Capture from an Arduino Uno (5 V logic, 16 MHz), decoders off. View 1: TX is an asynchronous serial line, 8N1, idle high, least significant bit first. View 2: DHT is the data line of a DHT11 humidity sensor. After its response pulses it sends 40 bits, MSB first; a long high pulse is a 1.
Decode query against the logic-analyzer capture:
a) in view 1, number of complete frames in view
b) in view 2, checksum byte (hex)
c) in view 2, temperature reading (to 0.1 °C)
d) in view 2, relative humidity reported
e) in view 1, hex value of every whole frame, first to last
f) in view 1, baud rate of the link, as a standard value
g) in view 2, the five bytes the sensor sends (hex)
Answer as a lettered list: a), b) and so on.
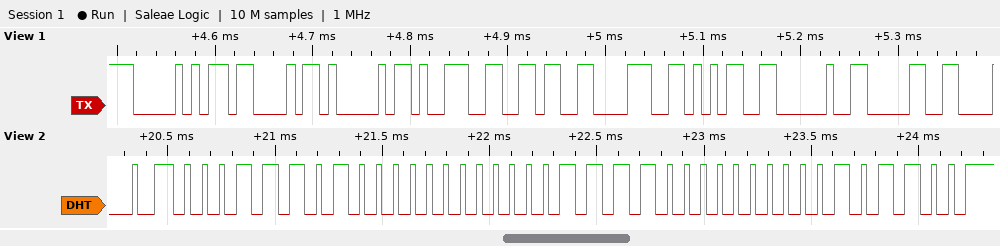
a) 9
b) 0x2C
c) 15.0 °C
d) 29 %
e) 50 43 41 39 36 38 35 20 30
f) 115200 baud
g) 1D 00 0F 00 2C
